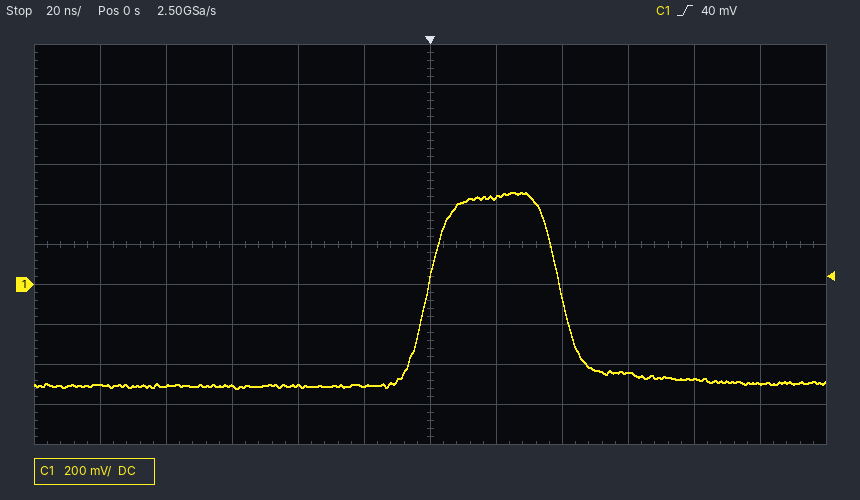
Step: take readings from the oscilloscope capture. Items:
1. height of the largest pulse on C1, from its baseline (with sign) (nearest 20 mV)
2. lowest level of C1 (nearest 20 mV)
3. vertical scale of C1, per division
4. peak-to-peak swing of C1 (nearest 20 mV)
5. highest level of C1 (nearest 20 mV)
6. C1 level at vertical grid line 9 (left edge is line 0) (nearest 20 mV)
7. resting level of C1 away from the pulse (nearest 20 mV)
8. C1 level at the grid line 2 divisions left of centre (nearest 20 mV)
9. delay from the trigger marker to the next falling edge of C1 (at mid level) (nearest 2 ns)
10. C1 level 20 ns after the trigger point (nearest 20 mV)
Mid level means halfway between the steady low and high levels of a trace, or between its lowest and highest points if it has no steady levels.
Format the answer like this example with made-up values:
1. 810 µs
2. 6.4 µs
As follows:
1. +960 mV
2. -520 mV
3. 200 mV
4. 980 mV
5. 460 mV
6. -440 mV
7. -500 mV
8. -500 mV
9. 40 ns
10. 440 mV
